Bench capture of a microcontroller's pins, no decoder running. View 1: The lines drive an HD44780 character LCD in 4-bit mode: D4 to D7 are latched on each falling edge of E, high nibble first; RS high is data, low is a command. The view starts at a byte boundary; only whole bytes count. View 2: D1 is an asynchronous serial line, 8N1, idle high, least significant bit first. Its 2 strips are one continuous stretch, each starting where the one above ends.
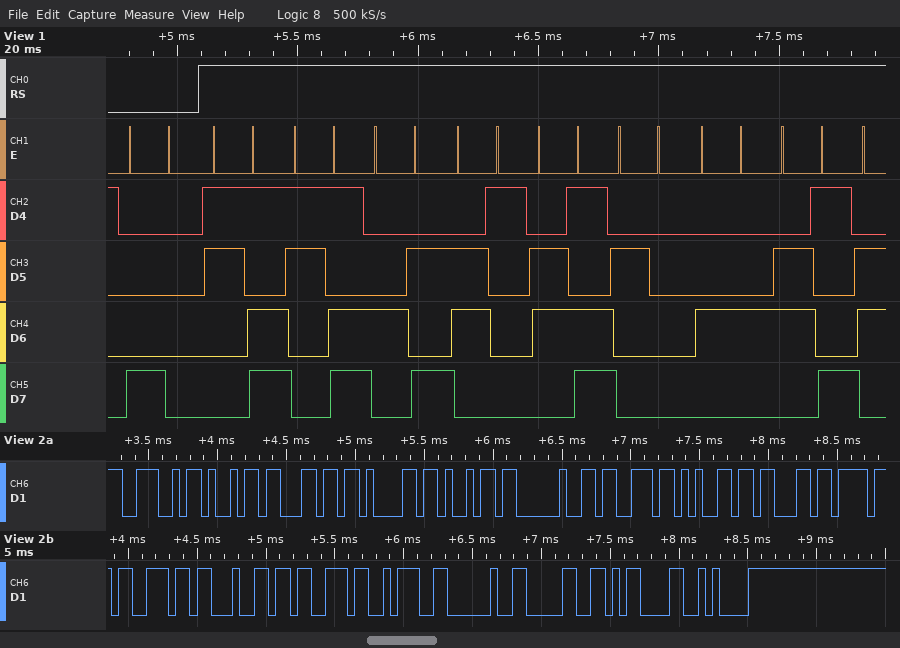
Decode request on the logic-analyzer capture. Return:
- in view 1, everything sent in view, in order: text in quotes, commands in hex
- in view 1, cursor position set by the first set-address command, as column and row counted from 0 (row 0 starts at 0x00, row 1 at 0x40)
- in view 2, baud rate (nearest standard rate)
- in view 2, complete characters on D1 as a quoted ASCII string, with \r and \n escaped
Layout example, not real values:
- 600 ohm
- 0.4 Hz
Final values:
- 0x80 "==Jam Di"
- column 0, row 0
- 19200 baud
- "Nilai seconds: 0\r\n"
